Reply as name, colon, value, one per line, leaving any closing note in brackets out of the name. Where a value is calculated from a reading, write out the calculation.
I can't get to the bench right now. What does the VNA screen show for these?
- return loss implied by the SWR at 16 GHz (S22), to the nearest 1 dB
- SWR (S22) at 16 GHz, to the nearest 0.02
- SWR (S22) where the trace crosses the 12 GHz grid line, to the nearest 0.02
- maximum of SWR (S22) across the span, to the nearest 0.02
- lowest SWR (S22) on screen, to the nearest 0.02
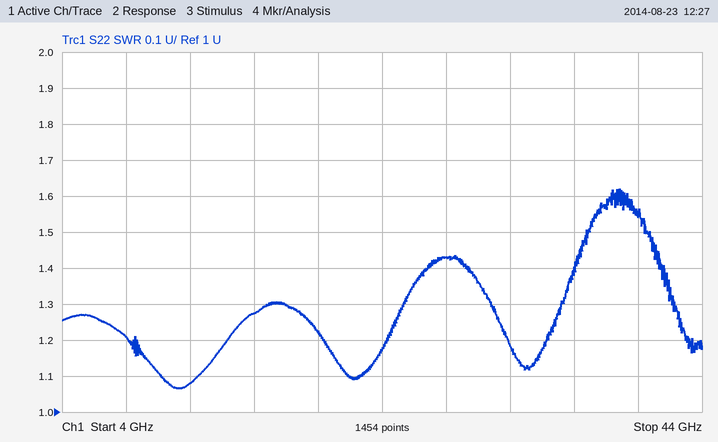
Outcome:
return loss implied by the SWR at 16 GHz (S22), to the nearest 1 dB: −20 log10((1.28 − 1)/(1.28 + 1)) ≈ 18 dB
SWR (S22) at 16 GHz, to the nearest 0.02: 1.28
SWR (S22) where the trace crosses the 12 GHz grid line, to the nearest 0.02: 1.08
maximum of SWR (S22) across the span, to the nearest 0.02: 1.62
lowest SWR (S22) on screen, to the nearest 0.02: 1.06
